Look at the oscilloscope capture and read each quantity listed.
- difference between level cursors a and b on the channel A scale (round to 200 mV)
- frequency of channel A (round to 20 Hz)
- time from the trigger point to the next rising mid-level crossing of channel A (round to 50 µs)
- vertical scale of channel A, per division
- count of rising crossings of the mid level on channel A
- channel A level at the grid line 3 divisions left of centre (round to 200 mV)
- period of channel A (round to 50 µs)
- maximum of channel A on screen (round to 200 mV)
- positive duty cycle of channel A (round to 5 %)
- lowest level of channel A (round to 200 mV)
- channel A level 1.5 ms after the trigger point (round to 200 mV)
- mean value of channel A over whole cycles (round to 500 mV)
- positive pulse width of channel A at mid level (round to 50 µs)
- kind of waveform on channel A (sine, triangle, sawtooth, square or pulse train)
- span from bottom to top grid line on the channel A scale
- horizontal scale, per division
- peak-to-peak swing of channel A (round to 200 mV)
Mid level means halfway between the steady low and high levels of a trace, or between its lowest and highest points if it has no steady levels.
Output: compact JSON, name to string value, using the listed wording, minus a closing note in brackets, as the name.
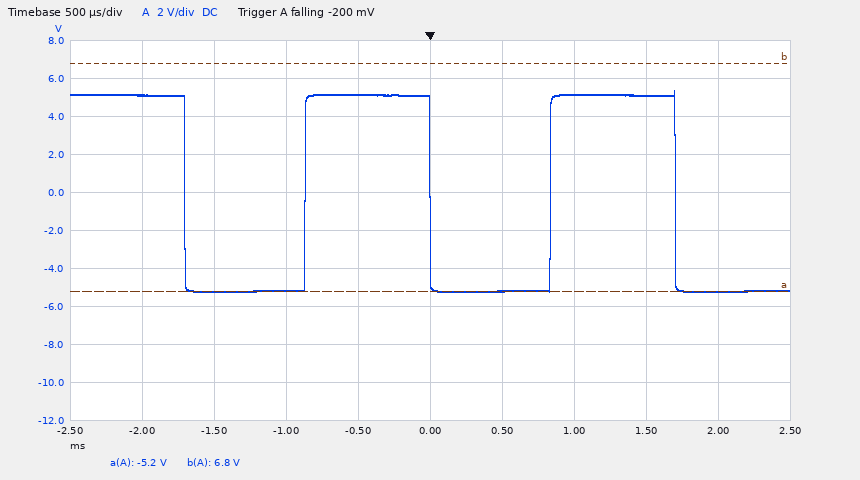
{"difference between level cursors a and b on the channel A scale": "12.0 V", "frequency of channel A": "580 Hz", "time from the trigger point to the next rising mid-level crossing of channel A": "850 µs", "vertical scale of channel A, per division": "2 V", "count of rising crossings of the mid level on channel A": "2", "channel A level at the grid line 3 divisions left of centre": "-5.2 V", "period of channel A": "1.70 ms", "maximum of channel A on screen": "5.4 V", "positive duty cycle of channel A": "50 %", "lowest level of channel A": "-5.2 V", "channel A level 1.5 ms after the trigger point": "5.2 V", "mean value of channel A over whole cycles": "0.0 V", "positive pulse width of channel A at mid level": "850 µs", "kind of waveform on channel A": "square", "span from bottom to top grid line on the channel A scale": "20 V", "horizontal scale, per division": "500 µs", "peak-to-peak swing of channel A": "10.6 V"}
